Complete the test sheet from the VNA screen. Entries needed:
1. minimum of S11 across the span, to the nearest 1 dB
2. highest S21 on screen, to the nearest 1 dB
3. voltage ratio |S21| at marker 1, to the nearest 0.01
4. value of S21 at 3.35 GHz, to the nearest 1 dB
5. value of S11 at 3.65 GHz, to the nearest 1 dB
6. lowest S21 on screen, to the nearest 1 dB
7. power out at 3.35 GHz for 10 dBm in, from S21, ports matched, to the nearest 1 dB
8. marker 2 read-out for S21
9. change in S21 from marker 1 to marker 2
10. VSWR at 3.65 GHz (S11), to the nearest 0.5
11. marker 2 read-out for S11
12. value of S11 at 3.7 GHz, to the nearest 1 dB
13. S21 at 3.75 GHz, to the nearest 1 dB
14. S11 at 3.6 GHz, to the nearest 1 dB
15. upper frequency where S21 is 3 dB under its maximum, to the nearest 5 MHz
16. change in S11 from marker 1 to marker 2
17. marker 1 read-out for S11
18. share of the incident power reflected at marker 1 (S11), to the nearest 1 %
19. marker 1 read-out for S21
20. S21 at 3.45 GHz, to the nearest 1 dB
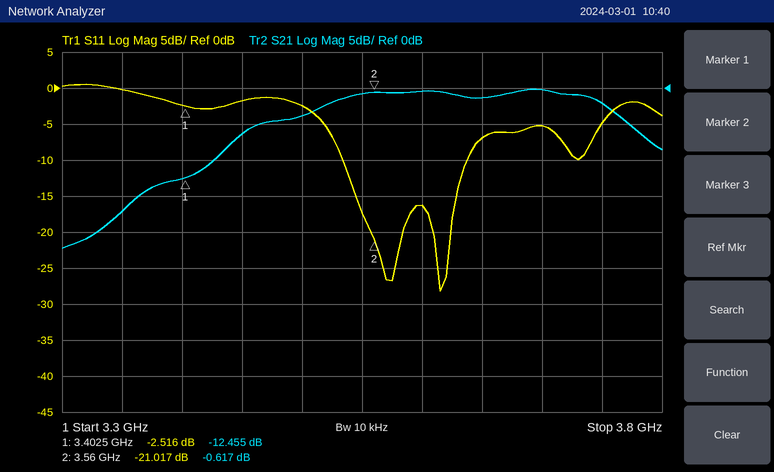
-28 dB
0 dB
0.24
-17 dB
-7 dB
-22 dB
-7 dBm
-0.617 dB
11.838 dB
2.5
-21.017 dB
-5 dB
-2 dB
-16 dB
3.760 GHz
-18.501 dB
-2.516 dB
56 %
-12.455 dB
-6 dB
